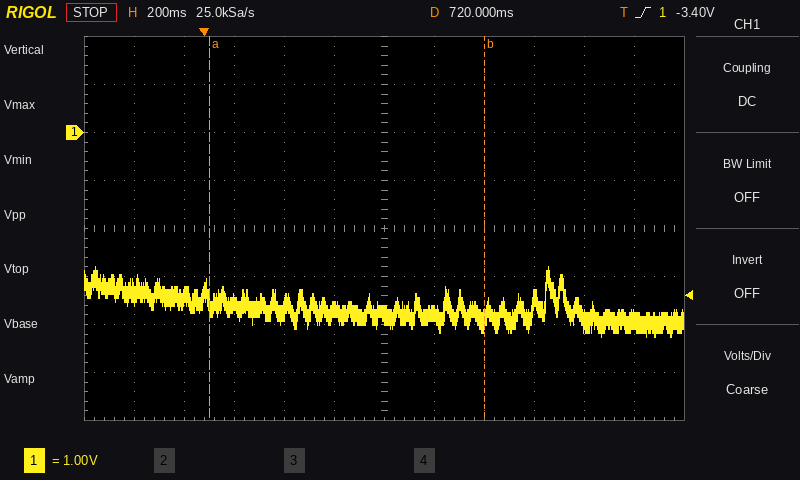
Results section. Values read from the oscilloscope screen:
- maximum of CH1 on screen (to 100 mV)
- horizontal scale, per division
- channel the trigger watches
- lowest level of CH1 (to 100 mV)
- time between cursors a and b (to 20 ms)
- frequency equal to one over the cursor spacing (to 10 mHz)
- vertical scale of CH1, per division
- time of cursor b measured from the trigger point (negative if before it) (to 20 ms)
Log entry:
-2.8 V
200 ms
CH1
-4.2 V
1.10 s
910 mHz
1 V
+1.12 s
